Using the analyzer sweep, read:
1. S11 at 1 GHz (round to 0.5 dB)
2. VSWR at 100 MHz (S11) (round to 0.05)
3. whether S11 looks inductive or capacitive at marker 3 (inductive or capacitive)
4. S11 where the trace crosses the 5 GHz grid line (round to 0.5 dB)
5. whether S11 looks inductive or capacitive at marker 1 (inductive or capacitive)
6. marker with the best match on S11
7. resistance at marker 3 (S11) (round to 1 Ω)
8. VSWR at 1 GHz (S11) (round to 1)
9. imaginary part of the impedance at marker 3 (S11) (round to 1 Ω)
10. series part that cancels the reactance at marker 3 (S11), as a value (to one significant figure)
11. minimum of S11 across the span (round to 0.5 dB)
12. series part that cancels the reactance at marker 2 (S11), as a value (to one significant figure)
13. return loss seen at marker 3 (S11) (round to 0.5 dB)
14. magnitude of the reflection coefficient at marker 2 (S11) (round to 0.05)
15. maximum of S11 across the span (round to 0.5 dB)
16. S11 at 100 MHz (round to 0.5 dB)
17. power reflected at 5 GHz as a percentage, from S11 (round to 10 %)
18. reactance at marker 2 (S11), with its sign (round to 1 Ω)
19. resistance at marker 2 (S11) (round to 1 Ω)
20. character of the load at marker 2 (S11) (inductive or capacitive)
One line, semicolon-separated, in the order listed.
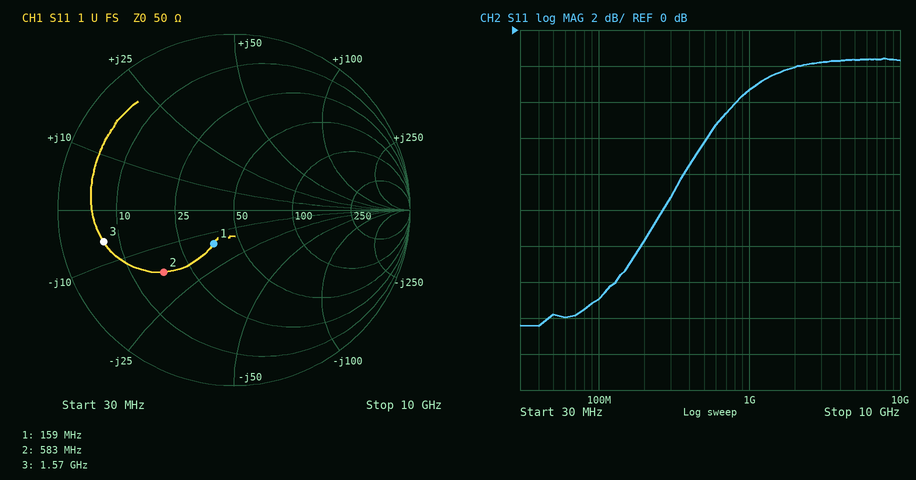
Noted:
-3.5 dB; 1.45; capacitive; -1.5 dB; capacitive; marker 1; 7 Ω; 5; -6 Ω; 600 pH; -16.5 dB; 5 nH; 2.5 dB; 0.55; -1.5 dB; -15.0 dB; 70 %; -17 Ω; 17 Ω; capacitive
